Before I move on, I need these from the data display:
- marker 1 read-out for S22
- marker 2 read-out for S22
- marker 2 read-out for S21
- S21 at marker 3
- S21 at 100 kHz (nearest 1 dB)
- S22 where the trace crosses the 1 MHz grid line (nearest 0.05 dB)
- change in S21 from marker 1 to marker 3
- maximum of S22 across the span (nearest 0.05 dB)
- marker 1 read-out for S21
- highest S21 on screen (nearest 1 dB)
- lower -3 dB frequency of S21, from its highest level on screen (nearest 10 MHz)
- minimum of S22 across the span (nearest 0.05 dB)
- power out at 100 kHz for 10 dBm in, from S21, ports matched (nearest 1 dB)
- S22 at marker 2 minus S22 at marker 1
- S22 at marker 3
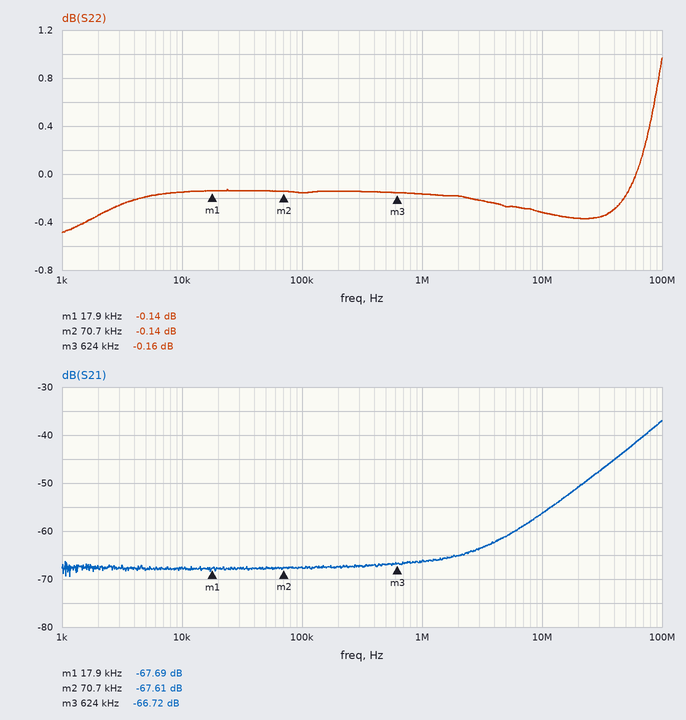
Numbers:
-0.14 dB
-0.14 dB
-67.61 dB
-66.72 dB
-68 dB
-0.15 dB
0.97 dB
0.95 dB
-67.69 dB
-37 dB
70 MHz
-0.50 dB
-58 dBm
0.00 dB
-0.16 dB
